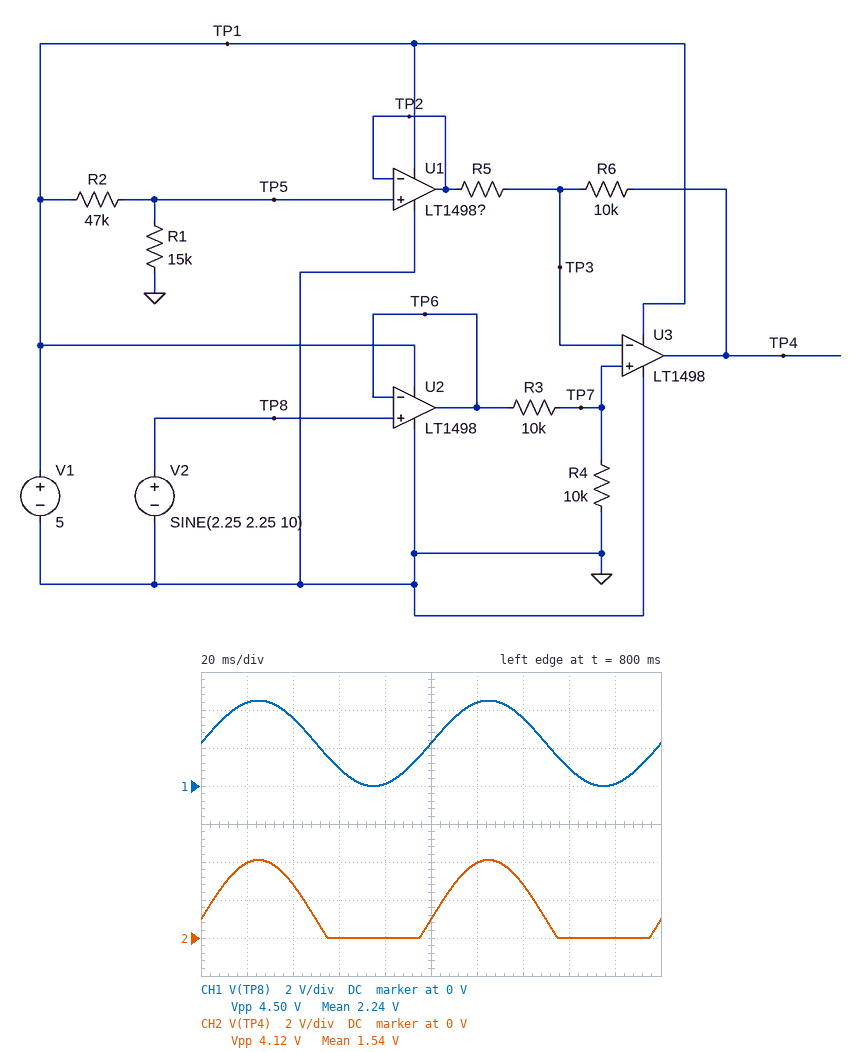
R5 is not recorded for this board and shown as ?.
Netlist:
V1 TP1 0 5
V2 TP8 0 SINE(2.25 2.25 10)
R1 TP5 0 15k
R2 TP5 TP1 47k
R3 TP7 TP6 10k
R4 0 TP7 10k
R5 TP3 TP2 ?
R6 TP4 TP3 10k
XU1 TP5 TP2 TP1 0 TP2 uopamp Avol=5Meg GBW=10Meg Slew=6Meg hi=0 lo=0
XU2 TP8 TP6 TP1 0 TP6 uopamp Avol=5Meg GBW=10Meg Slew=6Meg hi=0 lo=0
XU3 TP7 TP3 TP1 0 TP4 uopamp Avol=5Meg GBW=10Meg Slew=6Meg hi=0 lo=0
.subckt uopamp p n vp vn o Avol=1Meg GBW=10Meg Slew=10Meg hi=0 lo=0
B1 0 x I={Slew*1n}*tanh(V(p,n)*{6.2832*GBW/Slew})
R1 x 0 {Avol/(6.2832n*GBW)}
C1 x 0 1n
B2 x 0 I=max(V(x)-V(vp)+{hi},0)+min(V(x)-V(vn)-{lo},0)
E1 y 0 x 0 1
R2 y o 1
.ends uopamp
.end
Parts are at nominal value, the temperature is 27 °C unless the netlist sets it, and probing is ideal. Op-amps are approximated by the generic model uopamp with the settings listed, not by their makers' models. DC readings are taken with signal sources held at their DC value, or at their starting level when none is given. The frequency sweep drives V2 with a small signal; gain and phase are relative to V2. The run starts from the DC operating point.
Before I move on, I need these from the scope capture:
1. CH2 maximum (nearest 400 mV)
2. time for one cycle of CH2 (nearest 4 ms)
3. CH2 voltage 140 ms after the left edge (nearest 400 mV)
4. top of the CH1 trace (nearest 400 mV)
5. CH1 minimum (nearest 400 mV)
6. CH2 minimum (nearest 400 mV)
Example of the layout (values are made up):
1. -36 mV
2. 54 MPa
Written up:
1. 4.0 V
2. 100 ms
3. 2.8 V
4. 4.4 V
5. 0 V
6. 0 V
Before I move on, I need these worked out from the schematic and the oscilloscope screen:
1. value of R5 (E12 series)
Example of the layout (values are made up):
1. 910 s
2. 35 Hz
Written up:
1. 5.6 kΩ
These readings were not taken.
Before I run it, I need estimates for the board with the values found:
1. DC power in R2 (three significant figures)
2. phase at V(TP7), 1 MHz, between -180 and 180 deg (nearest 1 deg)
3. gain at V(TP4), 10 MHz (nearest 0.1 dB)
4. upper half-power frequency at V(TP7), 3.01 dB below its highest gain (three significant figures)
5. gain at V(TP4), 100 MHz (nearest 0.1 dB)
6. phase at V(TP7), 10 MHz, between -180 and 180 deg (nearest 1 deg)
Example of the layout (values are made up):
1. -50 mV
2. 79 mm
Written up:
1. 306 µW
2. -6 deg
3. -9.6 dB
4. 10.0 MHz
5. -46.1 dB
6. -45 deg
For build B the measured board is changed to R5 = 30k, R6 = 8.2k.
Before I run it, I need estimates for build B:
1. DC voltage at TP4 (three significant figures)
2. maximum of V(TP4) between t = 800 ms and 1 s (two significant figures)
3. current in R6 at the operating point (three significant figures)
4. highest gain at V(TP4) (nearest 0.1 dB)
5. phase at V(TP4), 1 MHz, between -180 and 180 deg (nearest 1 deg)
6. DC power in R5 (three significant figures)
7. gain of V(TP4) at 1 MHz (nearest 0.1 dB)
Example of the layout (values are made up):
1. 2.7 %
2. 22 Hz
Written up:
1. 1.10 V
2. 2.5 V
3. 2.82 µA
4. -3.9 dB
5. -13 deg
6. 239 nW
7. -4.0 dB
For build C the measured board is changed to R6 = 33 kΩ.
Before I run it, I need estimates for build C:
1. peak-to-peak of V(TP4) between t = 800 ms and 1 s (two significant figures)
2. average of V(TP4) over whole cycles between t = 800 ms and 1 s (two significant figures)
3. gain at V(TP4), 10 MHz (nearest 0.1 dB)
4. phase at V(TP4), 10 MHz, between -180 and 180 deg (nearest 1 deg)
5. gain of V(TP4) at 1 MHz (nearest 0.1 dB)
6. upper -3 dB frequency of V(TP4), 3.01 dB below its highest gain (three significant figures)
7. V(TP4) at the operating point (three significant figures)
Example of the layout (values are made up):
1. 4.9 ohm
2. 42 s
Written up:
1. 5.0 V
2. 2.1 V
3. -9.1 dB
4. -127 deg
5. 9.0 dB
6. 1.42 MHz
7. 626 mV
